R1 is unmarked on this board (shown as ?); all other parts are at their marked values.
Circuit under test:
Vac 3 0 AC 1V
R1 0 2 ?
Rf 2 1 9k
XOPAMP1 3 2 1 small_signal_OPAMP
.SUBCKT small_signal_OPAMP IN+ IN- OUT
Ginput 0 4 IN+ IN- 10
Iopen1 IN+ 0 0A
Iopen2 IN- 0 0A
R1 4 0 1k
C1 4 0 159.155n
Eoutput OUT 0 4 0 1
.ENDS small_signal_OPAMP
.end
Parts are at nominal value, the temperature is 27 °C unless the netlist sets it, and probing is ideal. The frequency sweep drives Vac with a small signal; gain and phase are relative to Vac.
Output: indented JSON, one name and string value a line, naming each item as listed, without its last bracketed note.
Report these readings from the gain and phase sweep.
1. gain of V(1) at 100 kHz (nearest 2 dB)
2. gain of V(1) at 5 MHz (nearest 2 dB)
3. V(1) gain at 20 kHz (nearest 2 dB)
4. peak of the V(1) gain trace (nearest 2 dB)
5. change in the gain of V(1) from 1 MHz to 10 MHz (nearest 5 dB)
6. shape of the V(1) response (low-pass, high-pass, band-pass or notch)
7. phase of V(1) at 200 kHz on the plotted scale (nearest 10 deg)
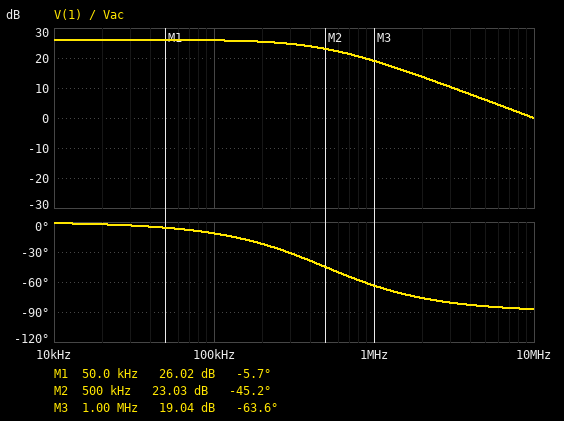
{
  "gain of V(1) at 100 kHz": "26 dB",
  "gain of V(1) at 5 MHz": "6 dB",
  "V(1) gain at 20 kHz": "26 dB",
  "peak of the V(1) gain trace": "26 dB",
  "change in the gain of V(1) from 1 MHz to 10 MHz": "-20 dB",
  "shape of the V(1) response": "low-pass",
  "phase of V(1) at 200 kHz on the plotted scale": "-20 deg"
}
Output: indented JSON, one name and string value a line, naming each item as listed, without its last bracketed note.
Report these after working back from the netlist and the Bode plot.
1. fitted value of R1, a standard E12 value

{
  "fitted value of R1, a standard E12 value": "470 Ω"
}
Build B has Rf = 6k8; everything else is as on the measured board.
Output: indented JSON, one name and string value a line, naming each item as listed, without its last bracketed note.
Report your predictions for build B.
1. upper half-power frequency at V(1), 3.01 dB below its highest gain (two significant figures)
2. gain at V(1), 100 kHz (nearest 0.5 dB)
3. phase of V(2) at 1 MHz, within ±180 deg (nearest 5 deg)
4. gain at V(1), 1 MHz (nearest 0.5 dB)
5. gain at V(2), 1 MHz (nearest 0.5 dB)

{
  "upper half-power frequency at V(1), 3.01 dB below its highest gain": "650 kHz",
  "gain at V(1), 100 kHz": "23.5 dB",
  "phase of V(2) at 1 MHz, within ±180 deg": "-55 deg",
  "gain at V(1), 1 MHz": "18.5 dB",
  "gain at V(2), 1 MHz": "-5.5 dB"
}
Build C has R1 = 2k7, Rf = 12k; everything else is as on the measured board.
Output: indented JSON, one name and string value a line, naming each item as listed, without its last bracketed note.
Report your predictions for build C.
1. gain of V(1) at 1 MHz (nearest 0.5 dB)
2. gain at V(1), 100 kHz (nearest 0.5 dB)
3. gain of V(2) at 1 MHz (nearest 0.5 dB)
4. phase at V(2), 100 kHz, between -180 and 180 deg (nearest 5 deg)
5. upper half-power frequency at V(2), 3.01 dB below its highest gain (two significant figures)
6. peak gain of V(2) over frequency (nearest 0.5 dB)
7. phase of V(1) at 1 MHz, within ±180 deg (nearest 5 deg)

{
  "gain of V(1) at 1 MHz": "13.5 dB",
  "gain at V(1), 100 kHz": "14.5 dB",
  "gain of V(2) at 1 MHz": "-1.0 dB",
  "phase at V(2), 100 kHz, between -180 and 180 deg": "-5 deg",
  "upper half-power frequency at V(2), 3.01 dB below its highest gain": "1.8 MHz",
  "peak gain of V(2) over frequency": "0 dB",
  "phase of V(1) at 1 MHz, within ±180 deg": "-30 deg"
}
